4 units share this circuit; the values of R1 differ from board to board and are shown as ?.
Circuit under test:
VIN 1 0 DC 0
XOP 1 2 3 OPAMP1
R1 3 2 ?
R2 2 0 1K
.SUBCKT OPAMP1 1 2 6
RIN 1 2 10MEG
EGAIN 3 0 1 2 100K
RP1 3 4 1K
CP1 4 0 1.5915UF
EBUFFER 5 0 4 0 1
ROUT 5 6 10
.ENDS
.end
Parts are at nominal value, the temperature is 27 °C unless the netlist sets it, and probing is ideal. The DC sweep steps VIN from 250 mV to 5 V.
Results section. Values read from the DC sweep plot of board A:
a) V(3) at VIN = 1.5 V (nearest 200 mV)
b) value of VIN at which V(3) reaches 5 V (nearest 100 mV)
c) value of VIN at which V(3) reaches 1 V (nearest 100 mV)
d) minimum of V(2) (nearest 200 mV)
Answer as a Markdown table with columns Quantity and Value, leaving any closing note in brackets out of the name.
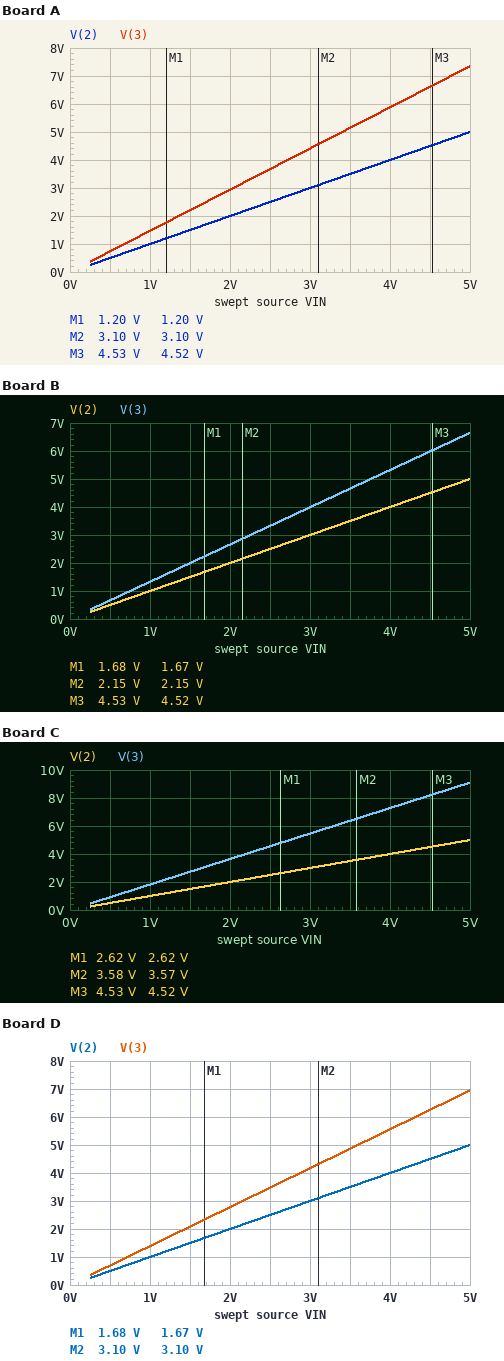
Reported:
| Quantity | Value |
|---|---|
| V(3) at VIN = 1.5 V | 2.2 V |
| value of VIN at which V(3) reaches 5 V | 3.4 V |
| value of VIN at which V(3) reaches 1 V | 700 mV |
| minimum of V(2) | 200 mV |
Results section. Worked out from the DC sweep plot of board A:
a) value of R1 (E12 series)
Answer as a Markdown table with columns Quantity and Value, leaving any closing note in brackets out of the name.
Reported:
| Quantity | Value |
|---|---|
| value of R1 | 470 Ω |
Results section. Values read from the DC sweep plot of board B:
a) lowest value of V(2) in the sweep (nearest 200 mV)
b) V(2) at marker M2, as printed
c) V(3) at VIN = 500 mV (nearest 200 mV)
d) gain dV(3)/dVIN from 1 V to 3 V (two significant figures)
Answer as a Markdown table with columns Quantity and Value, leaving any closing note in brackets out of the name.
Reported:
| Quantity | Value |
|---|---|
| lowest value of V(2) in the sweep | 200 mV |
| V(2) at marker M2, as printed | 2.15 V |
| V(3) at VIN = 500 mV | 600 mV |
| gain dV(3)/dVIN from 1 V to 3 V | 1.3 V/V |
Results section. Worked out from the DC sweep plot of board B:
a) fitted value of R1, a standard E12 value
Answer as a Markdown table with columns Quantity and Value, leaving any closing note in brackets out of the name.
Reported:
| Quantity | Value |
|---|---|
| fitted value of R1, a standard E12 value | 330 Ω |
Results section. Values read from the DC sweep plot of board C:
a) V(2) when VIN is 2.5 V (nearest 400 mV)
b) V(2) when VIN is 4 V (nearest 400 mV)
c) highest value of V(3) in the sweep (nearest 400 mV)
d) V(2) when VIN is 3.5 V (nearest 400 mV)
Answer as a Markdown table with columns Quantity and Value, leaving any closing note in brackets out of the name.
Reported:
| Quantity | Value |
|---|---|
| V(2) when VIN is 2.5 V | 2.4 V |
| V(2) when VIN is 4 V | 4.0 V |
| highest value of V(3) in the sweep | 9.2 V |
| V(2) when VIN is 3.5 V | 3.6 V |
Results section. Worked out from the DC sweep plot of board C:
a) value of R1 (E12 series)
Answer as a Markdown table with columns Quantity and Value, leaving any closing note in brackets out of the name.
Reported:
| Quantity | Value |
|---|---|
| value of R1 | 820 Ω |
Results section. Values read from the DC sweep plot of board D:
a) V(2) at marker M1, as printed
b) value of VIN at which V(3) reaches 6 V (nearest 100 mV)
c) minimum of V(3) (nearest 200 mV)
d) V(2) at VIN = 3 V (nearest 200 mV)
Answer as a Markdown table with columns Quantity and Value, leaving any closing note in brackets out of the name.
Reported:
| Quantity | Value |
|---|---|
| V(2) at marker M1, as printed | 1.67 V |
| value of VIN at which V(3) reaches 6 V | 4.3 V |
| minimum of V(3) | 400 mV |
| V(2) at VIN = 3 V | 3.0 V |
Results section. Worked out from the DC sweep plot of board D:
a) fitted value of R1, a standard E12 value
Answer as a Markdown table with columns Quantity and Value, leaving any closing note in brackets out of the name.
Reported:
| Quantity | Value |
|---|---|
| fitted value of R1, a standard E12 value | 390 Ω |
